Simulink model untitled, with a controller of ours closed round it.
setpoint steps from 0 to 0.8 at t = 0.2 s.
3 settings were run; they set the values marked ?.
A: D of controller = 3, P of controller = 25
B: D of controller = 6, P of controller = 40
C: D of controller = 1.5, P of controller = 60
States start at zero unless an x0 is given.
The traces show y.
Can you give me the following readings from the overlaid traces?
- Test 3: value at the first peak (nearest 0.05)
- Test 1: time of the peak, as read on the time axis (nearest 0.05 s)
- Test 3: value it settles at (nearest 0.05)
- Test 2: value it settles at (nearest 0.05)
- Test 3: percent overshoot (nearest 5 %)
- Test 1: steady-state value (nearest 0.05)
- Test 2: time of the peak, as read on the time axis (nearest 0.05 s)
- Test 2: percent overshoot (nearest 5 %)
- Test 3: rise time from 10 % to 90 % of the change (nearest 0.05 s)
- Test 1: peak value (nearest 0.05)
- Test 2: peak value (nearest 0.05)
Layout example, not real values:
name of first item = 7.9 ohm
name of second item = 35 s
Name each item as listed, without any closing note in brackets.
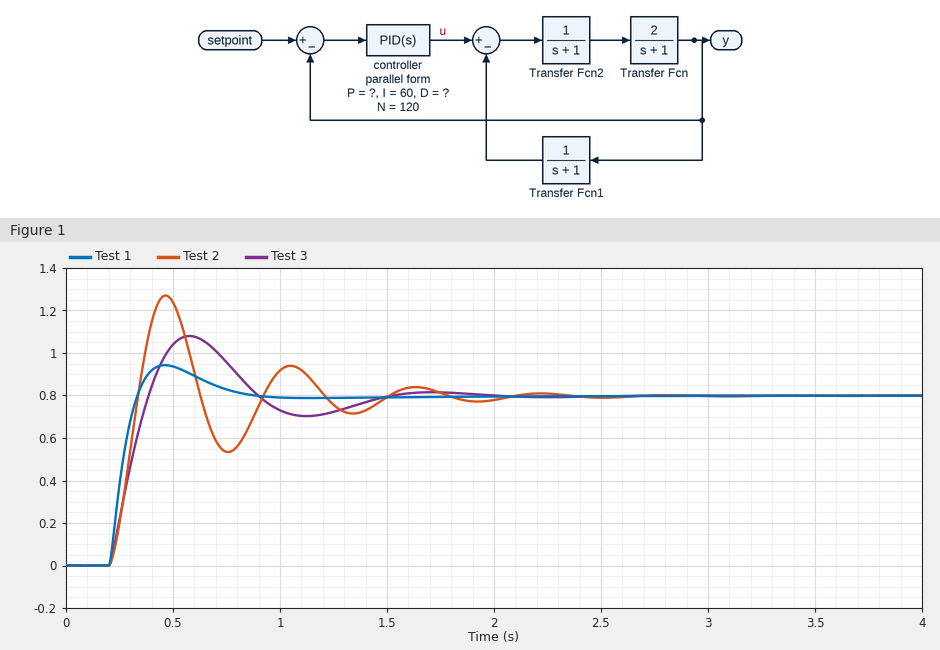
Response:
Test 3: value at the first peak = 1.10
Test 1: time of the peak, as read on the time axis = 0.45 s
Test 3: value it settles at = 0.80
Test 2: value it settles at = 0.80
Test 3: percent overshoot = 35 %
Test 1: steady-state value = 0.80
Test 2: time of the peak, as read on the time axis = 0.45 s
Test 2: percent overshoot = 60 %
Test 3: rise time from 10 % to 90 % of the change = 0.15 s
Test 1: peak value = 0.95
Test 2: peak value = 1.25
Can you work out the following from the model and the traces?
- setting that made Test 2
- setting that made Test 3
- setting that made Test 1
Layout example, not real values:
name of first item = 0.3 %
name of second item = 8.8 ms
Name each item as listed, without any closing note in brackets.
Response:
setting that made Test 2 = C
setting that made Test 3 = A
setting that made Test 1 = B
